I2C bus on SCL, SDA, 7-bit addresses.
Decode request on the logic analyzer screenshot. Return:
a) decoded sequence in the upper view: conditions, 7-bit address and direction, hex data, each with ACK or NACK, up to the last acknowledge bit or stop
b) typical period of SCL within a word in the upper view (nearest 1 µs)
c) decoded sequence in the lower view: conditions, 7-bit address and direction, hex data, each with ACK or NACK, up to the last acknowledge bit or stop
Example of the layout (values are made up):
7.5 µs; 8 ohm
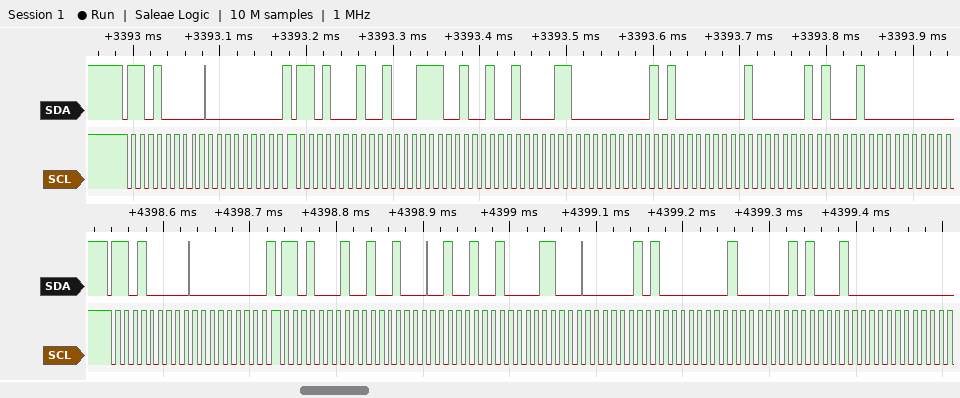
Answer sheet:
start, address 68 write ACK, 00 ACK, repeated start, address 68 read ACK, 47 ACK, 49 ACK, 18 ACK, 05 ACK, 01 ACK, 05 ACK, 20 ACK; 10 µs; start, address 68 write ACK, 00 ACK, repeated start, address 68 read ACK, 48 ACK, 49 ACK, 18 ACK, 05 ACK, 01 ACK, 05 ACK, 20 ACK
